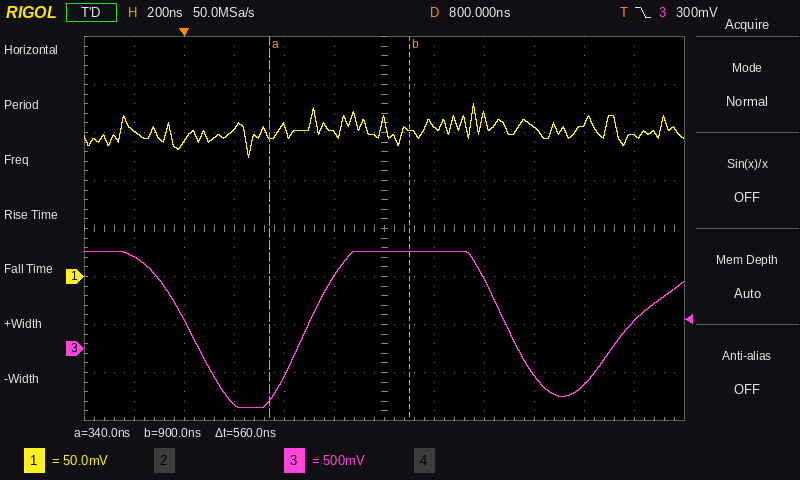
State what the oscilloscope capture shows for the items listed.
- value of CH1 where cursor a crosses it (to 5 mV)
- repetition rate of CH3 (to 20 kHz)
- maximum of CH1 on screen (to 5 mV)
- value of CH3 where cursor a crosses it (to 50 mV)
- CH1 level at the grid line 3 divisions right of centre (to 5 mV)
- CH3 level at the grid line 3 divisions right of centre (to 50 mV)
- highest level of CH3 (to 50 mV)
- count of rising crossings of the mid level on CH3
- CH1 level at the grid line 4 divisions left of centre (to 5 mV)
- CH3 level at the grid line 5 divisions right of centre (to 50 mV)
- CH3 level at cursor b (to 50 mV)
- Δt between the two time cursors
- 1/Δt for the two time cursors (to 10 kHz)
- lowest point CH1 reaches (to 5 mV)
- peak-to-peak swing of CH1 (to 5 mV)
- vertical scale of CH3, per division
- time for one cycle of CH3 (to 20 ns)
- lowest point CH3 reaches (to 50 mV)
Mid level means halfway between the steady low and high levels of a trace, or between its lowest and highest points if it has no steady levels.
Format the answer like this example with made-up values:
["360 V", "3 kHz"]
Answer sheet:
["145 mV", "780 kHz", "180 mV", "-550 mV", "155 mV", "-300 mV", "1.00 V", "2", "140 mV", "300 mV", "1.00 V", "560 ns", "1.79 MHz", "125 mV", "55 mV", "500 mV", "1.28 µs", "-600 mV"]
